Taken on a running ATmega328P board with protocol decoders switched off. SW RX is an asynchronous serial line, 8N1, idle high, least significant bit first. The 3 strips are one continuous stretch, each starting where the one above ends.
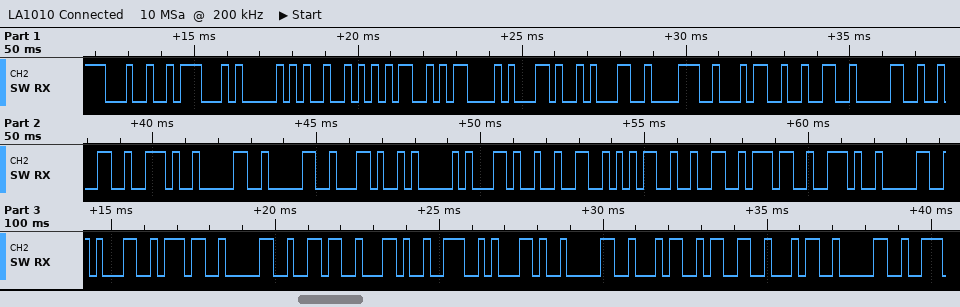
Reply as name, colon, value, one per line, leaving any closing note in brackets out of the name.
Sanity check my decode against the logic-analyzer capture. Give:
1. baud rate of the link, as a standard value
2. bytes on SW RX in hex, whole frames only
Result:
baud rate of the link, as a standard value: 4800 baud
bytes on SW RX in hex, whole frames only: 24 47 50 52 4D 43 2C 31 38 34 32 30 32 2E 30 30 2C 41 2C 32 35 32 37 2E 30 31 37 30 36 2C 4E 2C 30 34 33 34 30
